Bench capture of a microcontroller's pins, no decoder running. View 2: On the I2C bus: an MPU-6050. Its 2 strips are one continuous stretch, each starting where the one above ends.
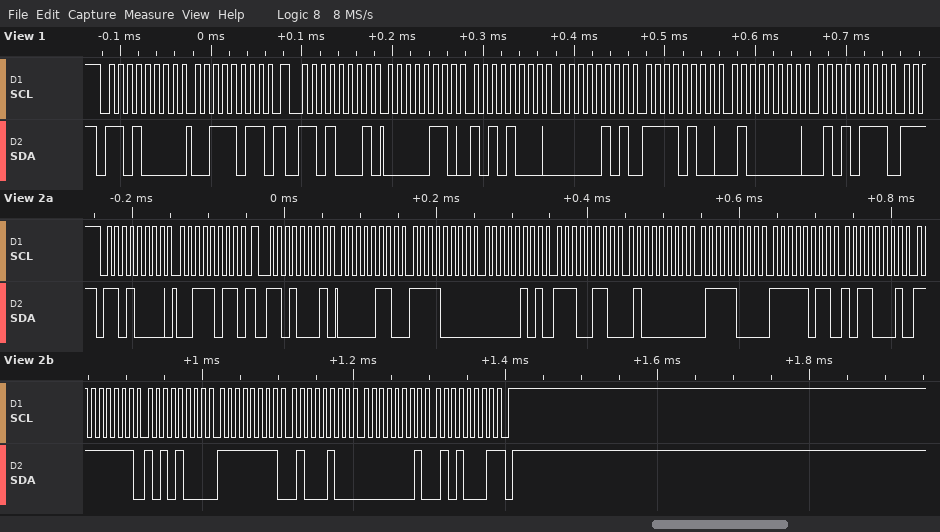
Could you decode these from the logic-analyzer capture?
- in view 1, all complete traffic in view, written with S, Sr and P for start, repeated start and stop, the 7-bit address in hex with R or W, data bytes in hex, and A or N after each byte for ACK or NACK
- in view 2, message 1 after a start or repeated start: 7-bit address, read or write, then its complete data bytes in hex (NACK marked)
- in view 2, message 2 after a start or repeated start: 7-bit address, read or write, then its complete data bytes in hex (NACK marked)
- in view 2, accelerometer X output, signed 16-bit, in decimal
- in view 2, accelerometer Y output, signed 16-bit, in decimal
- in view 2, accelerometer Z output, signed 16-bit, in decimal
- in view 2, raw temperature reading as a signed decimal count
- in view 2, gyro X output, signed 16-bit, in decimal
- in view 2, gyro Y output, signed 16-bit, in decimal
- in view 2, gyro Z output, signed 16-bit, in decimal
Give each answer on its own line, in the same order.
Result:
S 68W A 3B A Sr 68R A 06 A A8 A 05 A F4 A 40 A 57 A
0x68 write: 3B
0x68 read: 06 F0 05 E6 40 78 FB B1 FF A8 FF 44 01 51 NACK
1776
1510
16504
-1103
-88
-188
337
